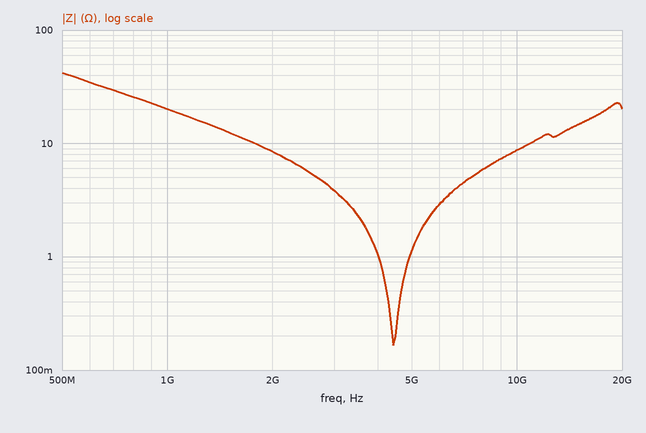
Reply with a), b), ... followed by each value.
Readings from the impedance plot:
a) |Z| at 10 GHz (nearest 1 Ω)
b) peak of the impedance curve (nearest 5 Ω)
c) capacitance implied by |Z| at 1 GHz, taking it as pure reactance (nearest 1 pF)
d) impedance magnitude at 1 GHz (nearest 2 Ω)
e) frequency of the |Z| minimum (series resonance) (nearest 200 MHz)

a) 9 Ω
b) 40 Ω
c) 8 pF
d) 20 Ω
e) 4.4 GHz
